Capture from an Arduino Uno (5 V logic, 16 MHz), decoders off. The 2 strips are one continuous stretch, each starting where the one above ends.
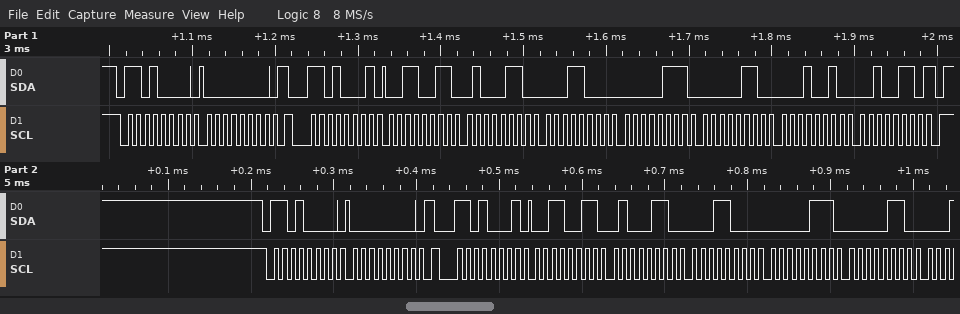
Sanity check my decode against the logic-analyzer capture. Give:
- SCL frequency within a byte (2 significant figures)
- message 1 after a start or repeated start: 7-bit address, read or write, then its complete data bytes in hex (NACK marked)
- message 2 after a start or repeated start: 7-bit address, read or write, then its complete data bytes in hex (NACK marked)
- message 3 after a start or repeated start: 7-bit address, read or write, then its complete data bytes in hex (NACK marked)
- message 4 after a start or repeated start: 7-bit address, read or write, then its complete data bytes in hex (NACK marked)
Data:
100 kHz
0x68 write: 00
0x68 read: 33 46 18 07 06 12 26 NACK
0x68 write: 00
0x68 read: 33 46 18 07 06
